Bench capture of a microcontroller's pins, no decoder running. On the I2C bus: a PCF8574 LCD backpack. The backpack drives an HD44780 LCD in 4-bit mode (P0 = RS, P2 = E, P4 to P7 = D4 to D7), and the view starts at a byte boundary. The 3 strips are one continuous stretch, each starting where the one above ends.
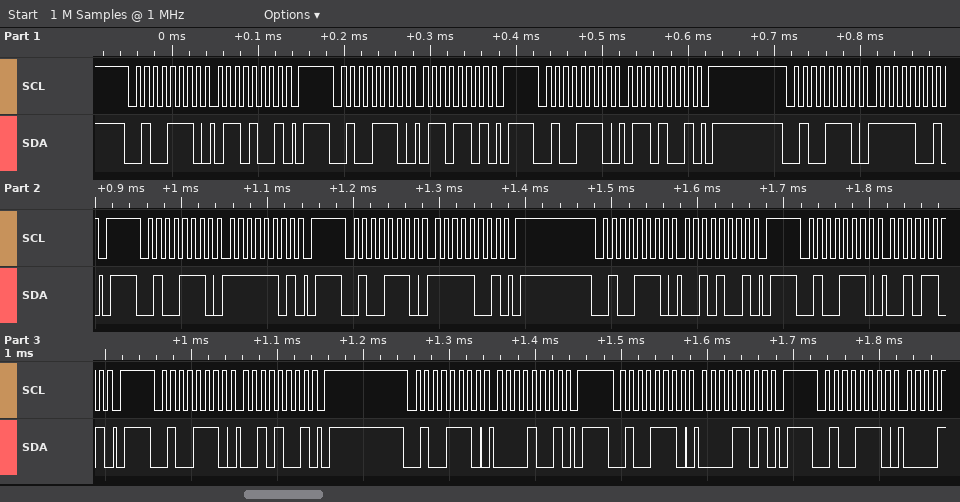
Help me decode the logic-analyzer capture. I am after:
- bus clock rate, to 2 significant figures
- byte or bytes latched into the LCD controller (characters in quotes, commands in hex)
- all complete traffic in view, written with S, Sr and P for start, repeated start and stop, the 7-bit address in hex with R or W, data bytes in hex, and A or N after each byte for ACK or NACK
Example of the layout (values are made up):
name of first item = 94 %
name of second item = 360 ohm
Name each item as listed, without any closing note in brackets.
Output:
bus clock rate, to 2 significant figures = 100 kHz
byte or bytes latched into the LCD controller = 'o'
all complete traffic in view, written with S, Sr and P for start, repeated start and stop, the 7-bit address in hex with R or W, data bytes in hex, and A or N after each byte for ACK or NACK = S 27W A 69 A P S 27W A 6D A P S 27W A 69 A P S 27W A F9 A P S 27W A FD A P S 27W A F9 A P S 27W A 29 A P S 27W A 2D A P S 27W A 29 A P S 27W A 09 A P S 27W A 0D A P S 27W A
